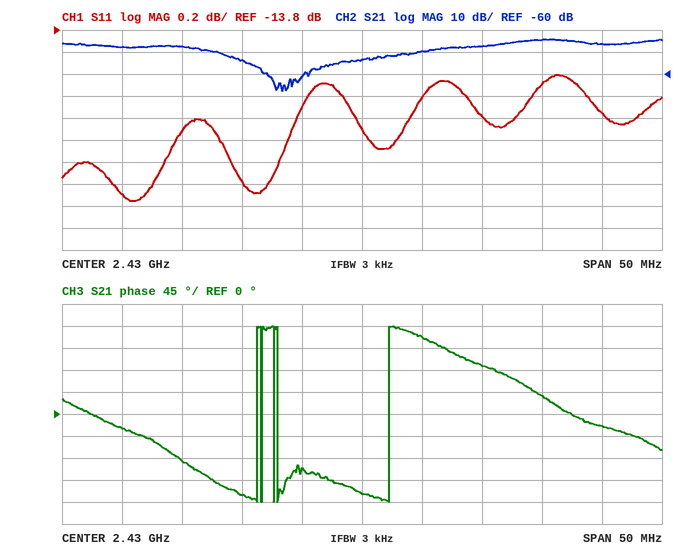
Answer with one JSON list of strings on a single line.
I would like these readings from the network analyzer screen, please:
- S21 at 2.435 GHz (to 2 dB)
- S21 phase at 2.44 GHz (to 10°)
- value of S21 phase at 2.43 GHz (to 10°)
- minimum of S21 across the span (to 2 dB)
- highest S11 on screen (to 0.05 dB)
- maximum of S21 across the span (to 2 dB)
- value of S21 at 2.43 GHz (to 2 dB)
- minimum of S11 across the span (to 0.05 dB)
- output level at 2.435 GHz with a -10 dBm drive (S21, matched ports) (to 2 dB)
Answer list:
["-50 dB", "100°", "-160°", "-68 dB", "-14.20 dB", "-44 dB", "-54 dB", "-15.35 dB", "-60 dBm"]
